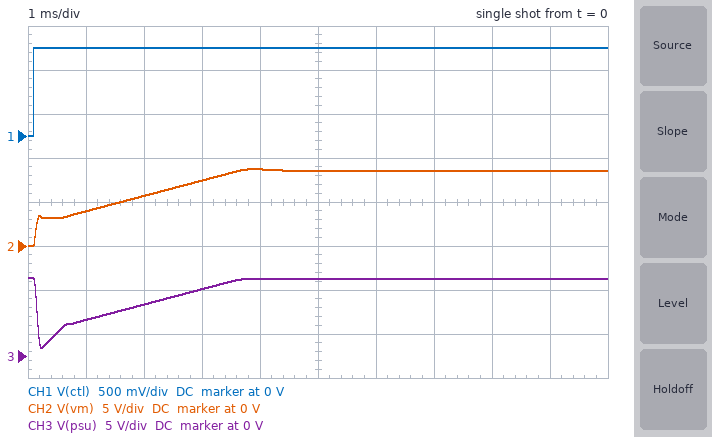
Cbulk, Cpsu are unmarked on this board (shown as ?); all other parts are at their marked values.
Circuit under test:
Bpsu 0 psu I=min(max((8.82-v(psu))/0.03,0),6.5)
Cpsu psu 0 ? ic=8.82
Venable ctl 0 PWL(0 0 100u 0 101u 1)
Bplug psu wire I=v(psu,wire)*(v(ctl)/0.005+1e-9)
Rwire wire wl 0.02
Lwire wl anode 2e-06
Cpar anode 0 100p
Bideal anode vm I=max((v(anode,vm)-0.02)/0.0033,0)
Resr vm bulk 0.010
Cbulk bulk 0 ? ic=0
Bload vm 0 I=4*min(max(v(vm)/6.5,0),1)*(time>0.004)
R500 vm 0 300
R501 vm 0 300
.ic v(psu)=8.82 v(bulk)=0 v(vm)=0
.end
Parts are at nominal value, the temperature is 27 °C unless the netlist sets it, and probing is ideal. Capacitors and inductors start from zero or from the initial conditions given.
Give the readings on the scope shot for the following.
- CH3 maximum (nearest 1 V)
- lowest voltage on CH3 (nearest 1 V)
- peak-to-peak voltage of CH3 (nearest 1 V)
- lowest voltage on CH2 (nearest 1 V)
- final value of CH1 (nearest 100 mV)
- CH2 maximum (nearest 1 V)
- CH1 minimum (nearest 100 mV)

9 V
1 V
8 V
0 V
1.0 V
9 V
0 V
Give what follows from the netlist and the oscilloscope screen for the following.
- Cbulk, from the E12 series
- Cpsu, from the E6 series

2.7 mF
1 mF
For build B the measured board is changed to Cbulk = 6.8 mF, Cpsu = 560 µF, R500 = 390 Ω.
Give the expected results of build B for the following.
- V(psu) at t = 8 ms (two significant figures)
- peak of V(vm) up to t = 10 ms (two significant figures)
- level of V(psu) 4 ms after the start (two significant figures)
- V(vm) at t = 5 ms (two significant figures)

6.1 V
6.6 V
4.3 V
4.6 V
